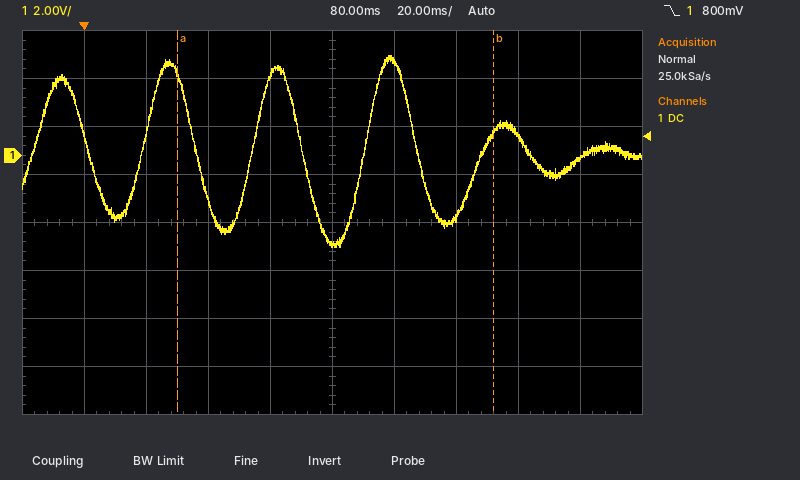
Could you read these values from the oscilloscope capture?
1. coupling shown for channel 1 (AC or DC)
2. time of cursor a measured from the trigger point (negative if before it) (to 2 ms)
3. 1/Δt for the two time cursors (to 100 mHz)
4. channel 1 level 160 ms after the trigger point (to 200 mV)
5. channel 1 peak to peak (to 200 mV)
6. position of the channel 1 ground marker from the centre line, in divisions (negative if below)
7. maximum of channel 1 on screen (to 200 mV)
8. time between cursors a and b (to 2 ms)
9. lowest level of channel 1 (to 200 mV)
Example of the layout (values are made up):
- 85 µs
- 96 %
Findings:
- DC
- +30 ms
- 9.8 Hz
- -200 mV
- 8.0 V
- +1.4 div
- 4.2 V
- 102 ms
- -3.8 V
